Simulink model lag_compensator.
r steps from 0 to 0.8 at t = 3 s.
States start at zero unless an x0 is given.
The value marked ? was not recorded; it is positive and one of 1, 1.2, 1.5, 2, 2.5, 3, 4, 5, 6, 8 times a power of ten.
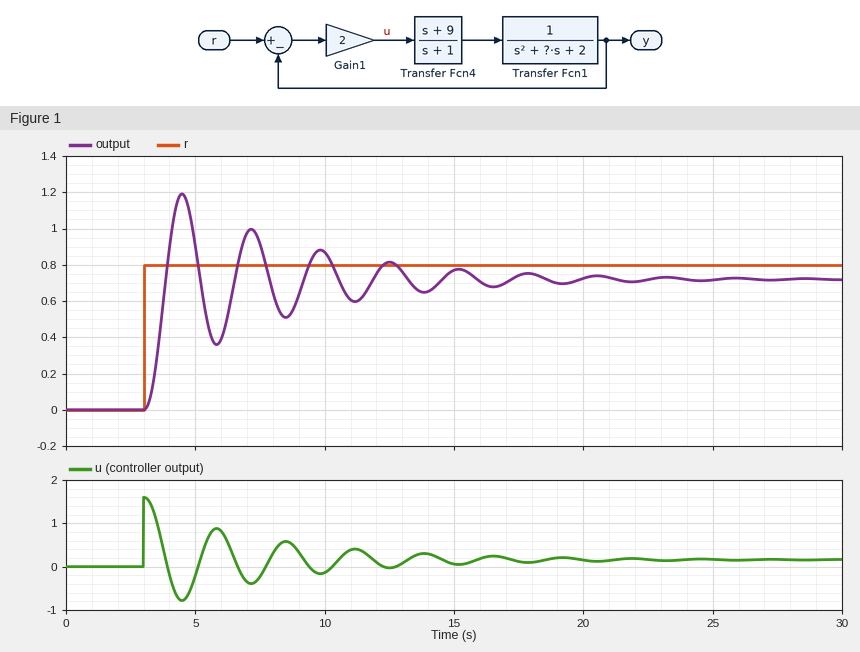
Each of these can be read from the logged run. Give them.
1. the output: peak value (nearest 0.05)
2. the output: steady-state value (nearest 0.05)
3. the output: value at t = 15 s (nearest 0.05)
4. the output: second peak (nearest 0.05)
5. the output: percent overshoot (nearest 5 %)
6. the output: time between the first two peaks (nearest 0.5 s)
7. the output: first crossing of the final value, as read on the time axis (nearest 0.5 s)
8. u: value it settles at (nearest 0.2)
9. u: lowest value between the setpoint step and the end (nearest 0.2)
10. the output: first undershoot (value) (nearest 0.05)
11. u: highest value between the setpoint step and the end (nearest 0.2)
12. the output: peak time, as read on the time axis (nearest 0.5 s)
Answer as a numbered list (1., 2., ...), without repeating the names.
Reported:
1. 1.20
2. 0.70
3. 0.75
4. 1.00
5. 65 %
6. 2.5 s
7. 4.0 s
8. 0.2
9. -0.8
10. 0.35
11. 1.6
12. 4.5 s
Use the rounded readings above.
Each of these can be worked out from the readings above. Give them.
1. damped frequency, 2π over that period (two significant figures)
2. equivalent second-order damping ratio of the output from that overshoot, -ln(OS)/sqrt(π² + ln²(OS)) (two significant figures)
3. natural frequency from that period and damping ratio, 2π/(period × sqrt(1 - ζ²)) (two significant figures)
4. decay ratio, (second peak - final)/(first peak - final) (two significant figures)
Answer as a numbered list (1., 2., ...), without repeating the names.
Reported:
1. 2.5 rad/s
2. 0.14
3. 2.5 rad/s
4. 0.60
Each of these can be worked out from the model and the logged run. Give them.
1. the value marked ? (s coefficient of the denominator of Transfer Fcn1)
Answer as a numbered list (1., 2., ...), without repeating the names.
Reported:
1. 3
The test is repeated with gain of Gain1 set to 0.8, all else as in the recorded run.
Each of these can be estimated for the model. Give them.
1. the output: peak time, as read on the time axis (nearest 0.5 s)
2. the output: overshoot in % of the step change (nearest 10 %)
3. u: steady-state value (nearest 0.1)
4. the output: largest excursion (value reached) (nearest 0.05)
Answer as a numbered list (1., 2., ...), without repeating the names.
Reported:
1. 5.0 s
2. 40 %
3. 0.1
4. 0.85
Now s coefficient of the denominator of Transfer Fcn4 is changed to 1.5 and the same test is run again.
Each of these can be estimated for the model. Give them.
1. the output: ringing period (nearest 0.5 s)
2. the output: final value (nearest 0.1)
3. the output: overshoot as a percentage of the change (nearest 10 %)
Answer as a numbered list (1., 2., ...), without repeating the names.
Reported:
1. 3.0 s
2. 0.7
3. 60 %
